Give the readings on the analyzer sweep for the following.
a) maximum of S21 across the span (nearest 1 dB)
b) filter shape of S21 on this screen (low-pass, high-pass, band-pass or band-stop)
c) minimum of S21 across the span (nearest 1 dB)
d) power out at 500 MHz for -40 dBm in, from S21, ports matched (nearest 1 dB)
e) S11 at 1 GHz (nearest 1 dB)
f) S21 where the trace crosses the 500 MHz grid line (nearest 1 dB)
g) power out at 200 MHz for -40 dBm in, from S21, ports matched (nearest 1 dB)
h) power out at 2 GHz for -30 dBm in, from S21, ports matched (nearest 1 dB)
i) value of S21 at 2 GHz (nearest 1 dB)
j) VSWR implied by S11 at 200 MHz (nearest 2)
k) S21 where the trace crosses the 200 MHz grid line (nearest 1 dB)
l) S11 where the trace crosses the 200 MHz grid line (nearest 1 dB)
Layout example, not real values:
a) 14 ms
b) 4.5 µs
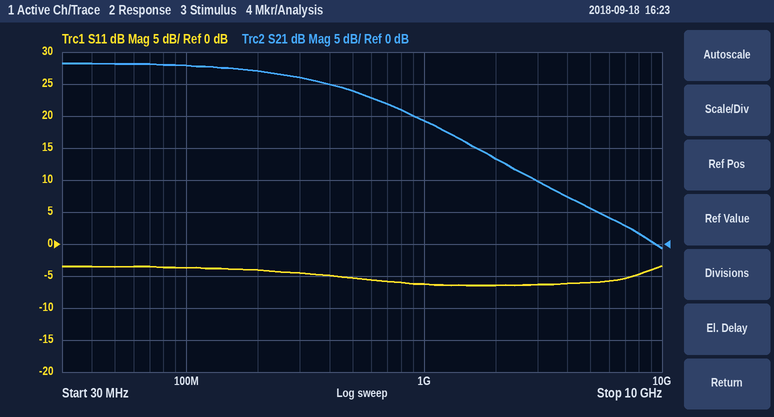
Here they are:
a) 28 dB
b) low-pass
c) -1 dB
d) -16 dBm
e) -6 dB
f) 24 dB
g) -13 dBm
h) -17 dBm
i) 13 dB
j) 4
k) 27 dB
l) -4 dB
